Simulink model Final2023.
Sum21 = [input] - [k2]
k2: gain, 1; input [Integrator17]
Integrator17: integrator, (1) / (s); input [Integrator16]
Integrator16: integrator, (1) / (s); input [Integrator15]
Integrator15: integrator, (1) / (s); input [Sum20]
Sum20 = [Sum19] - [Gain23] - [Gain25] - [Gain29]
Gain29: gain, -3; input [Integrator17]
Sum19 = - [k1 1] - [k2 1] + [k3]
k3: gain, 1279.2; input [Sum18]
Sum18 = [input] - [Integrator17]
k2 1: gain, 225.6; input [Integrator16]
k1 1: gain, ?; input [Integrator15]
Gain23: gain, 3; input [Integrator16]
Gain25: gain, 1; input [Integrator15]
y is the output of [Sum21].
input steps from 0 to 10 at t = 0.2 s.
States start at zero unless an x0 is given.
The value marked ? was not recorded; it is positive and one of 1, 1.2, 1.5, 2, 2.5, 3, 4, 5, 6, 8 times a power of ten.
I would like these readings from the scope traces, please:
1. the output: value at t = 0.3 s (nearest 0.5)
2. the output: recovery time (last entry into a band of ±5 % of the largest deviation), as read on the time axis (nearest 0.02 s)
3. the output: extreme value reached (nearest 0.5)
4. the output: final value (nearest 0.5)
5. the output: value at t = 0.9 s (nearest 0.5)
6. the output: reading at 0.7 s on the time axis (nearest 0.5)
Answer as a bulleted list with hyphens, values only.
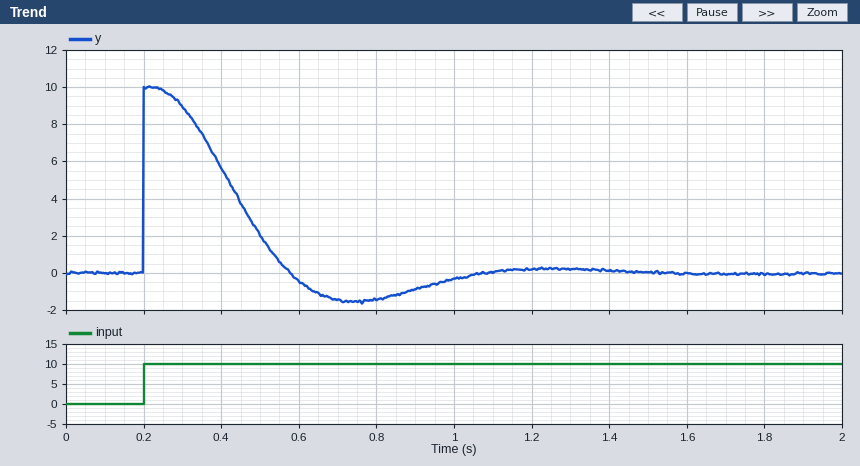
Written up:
- 9.0
- 0.96 s
- 10.0
- 0.0
- -1.0
- -1.5
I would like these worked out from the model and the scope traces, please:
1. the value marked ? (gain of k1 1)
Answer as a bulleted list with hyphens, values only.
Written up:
- 30
